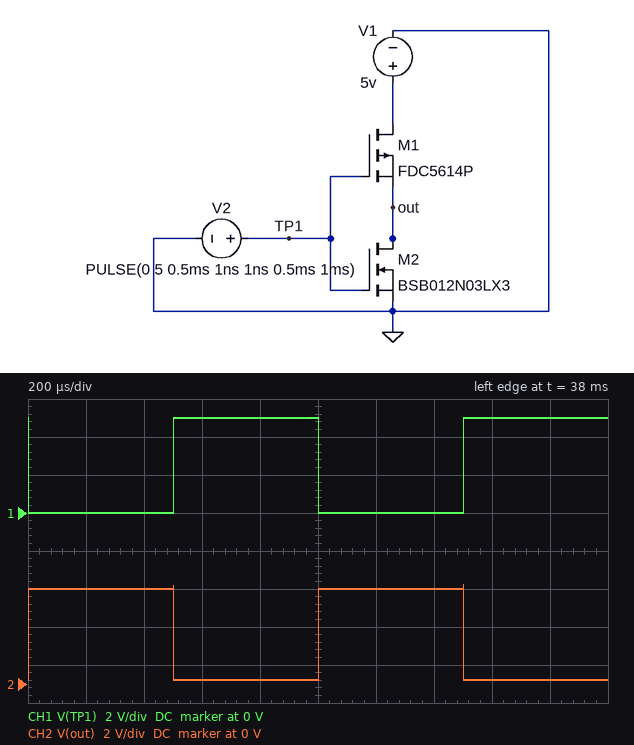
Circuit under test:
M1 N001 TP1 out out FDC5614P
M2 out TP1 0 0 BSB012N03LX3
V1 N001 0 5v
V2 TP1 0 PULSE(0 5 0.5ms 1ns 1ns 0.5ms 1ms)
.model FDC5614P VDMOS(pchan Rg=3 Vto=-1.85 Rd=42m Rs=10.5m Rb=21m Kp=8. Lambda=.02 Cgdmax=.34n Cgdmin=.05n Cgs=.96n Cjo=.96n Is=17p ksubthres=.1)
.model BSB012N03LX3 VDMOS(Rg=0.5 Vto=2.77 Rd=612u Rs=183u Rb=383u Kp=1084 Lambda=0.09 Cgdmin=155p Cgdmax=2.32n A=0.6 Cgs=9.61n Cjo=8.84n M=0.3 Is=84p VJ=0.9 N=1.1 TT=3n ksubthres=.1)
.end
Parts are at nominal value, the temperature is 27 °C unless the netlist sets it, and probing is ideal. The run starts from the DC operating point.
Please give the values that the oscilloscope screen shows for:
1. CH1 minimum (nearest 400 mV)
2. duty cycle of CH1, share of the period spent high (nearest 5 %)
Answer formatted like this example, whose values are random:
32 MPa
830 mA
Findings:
0 V
50 %
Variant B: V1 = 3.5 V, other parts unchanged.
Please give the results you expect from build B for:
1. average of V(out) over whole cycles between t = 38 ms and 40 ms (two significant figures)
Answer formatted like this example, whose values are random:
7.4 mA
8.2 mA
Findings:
1.8 V
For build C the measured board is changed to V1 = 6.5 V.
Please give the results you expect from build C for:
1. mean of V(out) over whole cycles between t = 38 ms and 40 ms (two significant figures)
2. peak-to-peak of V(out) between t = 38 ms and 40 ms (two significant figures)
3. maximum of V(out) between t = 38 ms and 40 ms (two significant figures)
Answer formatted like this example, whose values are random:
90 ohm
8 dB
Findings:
3.4 V
6.3 V
6.6 V
